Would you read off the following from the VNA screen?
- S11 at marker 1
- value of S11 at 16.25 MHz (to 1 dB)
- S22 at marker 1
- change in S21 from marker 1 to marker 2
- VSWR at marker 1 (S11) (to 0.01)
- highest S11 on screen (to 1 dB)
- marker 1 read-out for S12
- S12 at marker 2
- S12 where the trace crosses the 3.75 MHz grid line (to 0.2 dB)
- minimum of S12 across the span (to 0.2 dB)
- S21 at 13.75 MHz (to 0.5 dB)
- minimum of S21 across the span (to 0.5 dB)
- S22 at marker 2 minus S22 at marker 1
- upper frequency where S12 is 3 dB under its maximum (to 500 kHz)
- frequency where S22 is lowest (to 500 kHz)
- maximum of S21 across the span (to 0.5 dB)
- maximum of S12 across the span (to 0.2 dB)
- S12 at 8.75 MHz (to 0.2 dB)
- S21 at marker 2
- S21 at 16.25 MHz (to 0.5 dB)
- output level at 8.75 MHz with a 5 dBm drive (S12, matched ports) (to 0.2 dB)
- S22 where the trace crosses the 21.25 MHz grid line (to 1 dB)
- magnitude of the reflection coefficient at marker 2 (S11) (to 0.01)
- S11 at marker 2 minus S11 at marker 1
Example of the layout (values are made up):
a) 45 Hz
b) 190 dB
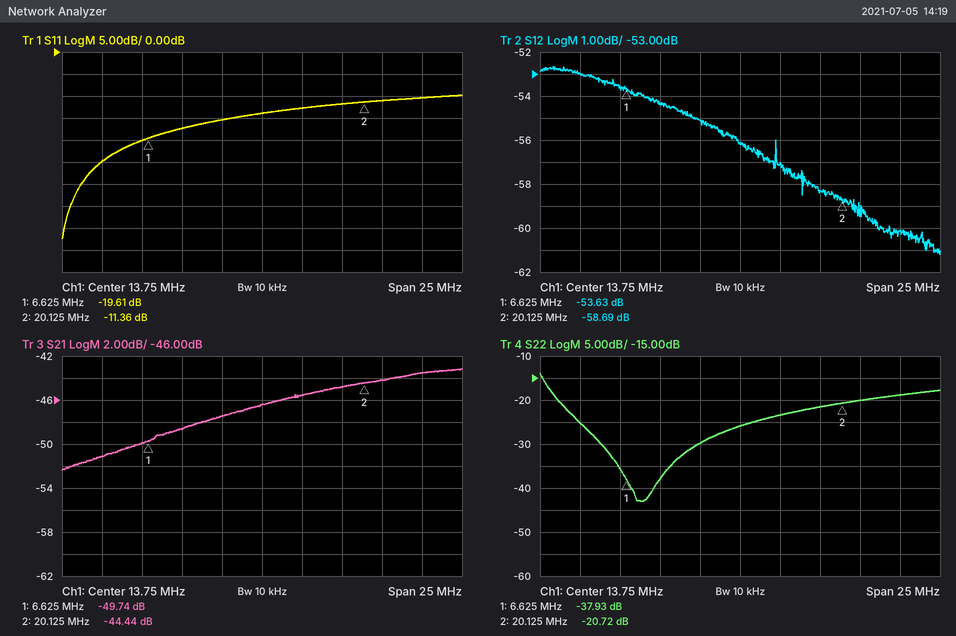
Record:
a) -19.61 dB
b) -13 dB
c) -37.93 dB
d) 5.30 dB
e) 1.23
f) -10 dB
g) -53.63 dB
h) -58.69 dB
i) -53.0 dB
j) -61.2 dB
k) -46.5 dB
l) -52.5 dB
m) 17.21 dB
n) 12.5 MHz
o) 7.5 MHz
p) -43.0 dB
q) -52.6 dB
r) -54.4 dB
s) -44.44 dB
t) -45.5 dB
u) -49.4 dBm
v) -20 dB
w) 0.27
x) 8.25 dB
